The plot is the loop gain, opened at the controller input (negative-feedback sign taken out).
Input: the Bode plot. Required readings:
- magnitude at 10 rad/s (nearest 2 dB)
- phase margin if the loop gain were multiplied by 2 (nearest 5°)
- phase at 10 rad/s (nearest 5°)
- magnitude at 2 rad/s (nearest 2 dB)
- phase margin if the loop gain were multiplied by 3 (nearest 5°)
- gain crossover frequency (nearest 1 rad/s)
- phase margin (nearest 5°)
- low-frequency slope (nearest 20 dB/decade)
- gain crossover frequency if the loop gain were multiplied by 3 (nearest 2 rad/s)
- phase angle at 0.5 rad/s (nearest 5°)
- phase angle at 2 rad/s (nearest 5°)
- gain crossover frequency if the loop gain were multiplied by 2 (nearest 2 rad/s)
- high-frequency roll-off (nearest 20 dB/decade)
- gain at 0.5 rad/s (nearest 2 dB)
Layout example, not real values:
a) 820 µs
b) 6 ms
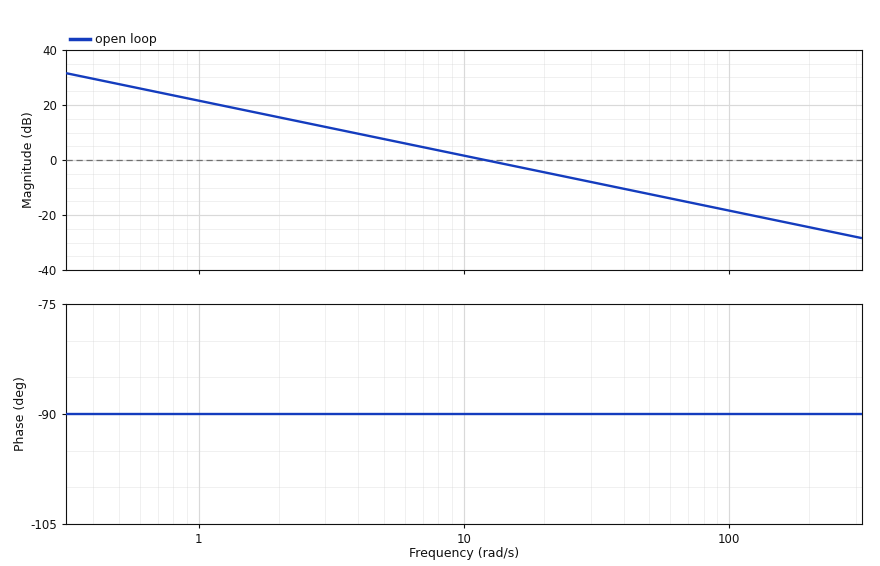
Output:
a) 2 dB
b) 90°
c) -90°
d) 16 dB
e) 90°
f) 12 rad/s
g) 90°
h) -20 dB/decade
i) 36 rad/s
j) -90°
k) -90°
l) 24 rad/s
m) -20 dB/decade
n) 28 dB
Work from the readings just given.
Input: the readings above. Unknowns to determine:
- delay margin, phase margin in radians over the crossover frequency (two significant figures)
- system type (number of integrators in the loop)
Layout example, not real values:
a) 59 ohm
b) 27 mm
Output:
a) 0.13 s
b) 1
